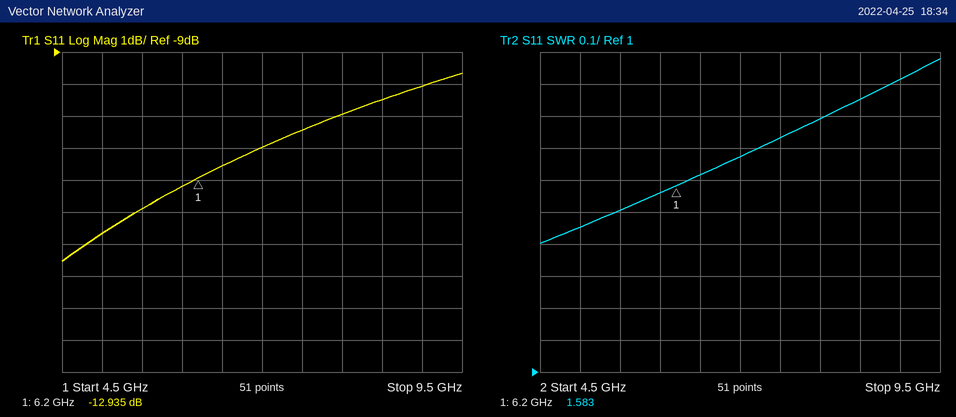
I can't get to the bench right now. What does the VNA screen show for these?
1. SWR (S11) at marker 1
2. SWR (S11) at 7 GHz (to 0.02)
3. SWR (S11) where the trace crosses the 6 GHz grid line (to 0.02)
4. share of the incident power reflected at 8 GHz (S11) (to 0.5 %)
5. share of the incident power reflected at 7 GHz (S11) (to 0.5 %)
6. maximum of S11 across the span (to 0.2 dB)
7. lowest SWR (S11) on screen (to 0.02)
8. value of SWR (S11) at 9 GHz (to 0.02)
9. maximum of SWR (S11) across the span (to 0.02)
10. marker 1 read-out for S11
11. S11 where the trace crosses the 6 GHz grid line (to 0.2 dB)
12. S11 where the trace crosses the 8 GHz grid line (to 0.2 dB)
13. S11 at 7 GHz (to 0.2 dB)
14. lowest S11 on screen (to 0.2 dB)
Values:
1.583
1.68
1.56
8.0 %
6.5 %
-9.6 dB
1.40
1.92
1.98
-12.935 dB
-13.2 dB
-11.0 dB
-12.0 dB
-15.6 dB
